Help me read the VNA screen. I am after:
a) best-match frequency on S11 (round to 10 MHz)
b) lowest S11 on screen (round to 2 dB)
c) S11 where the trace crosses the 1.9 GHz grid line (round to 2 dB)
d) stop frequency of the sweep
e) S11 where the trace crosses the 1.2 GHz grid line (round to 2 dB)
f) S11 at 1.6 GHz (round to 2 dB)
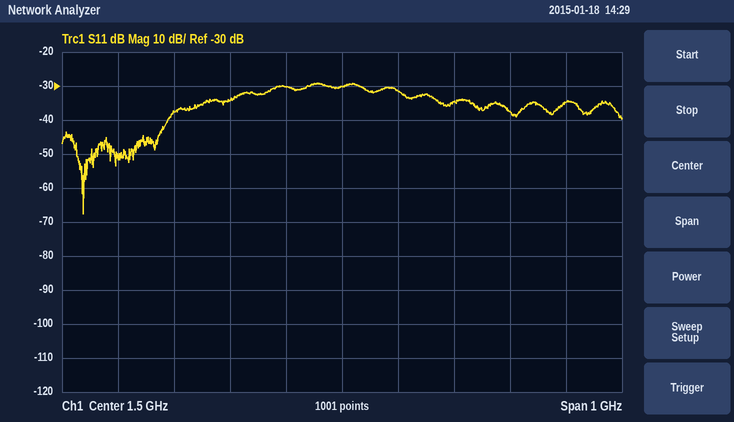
1.04 GHz
-68 dB
-34 dB
2 GHz
-38 dB
-32 dB
